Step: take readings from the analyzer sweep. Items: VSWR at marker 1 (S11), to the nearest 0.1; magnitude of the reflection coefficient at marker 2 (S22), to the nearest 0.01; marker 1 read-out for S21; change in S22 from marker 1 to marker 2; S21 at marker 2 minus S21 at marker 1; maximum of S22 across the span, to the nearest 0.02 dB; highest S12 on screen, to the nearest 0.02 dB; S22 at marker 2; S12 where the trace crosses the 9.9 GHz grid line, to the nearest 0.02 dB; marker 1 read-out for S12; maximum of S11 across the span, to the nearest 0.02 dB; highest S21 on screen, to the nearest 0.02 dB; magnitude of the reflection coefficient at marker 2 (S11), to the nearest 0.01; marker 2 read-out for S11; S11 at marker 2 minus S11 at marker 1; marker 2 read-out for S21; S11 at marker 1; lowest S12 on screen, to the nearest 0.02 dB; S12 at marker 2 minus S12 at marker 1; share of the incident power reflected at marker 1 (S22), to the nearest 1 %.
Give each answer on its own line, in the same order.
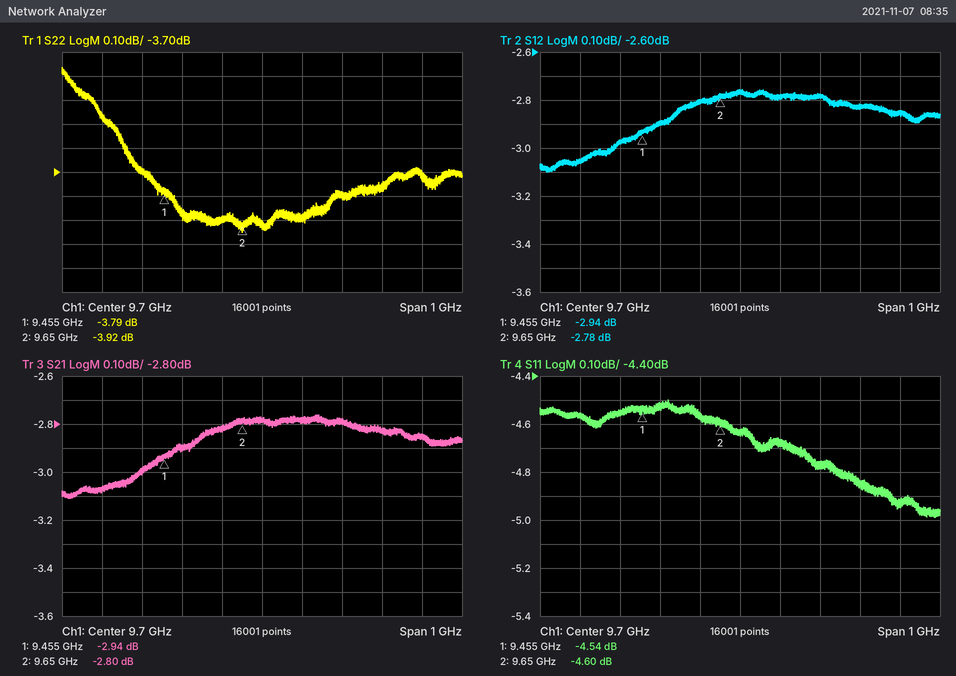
3.9
0.64
-2.94 dB
-0.13 dB
0.14 dB
-3.26 dB
-2.76 dB
-3.92 dB
-2.78 dB
-2.94 dB
-4.50 dB
-2.76 dB
0.59
-4.60 dB
-0.06 dB
-2.80 dB
-4.54 dB
-3.10 dB
0.16 dB
42 %
